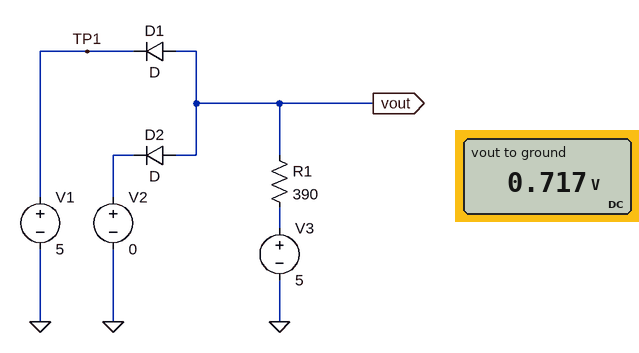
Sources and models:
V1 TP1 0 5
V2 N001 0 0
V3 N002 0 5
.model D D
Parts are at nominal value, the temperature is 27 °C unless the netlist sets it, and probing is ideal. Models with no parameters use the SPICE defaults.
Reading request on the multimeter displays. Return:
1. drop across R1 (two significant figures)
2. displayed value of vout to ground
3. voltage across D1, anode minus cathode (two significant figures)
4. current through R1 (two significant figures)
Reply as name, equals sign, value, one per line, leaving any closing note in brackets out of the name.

drop across R1 = 4.3 V
displayed value of vout to ground = 0.717 V
voltage across D1, anode minus cathode = -4.3 V
current through R1 = 11 mA
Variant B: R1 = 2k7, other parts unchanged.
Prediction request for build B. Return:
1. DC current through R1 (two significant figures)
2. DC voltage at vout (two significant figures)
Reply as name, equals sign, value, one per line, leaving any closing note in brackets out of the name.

DC current through R1 = 1.6 mA
DC voltage at vout = 670 mV
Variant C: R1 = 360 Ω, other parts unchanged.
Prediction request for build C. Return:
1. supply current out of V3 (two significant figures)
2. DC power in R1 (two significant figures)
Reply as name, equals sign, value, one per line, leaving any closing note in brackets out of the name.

supply current out of V3 = 12 mA
DC power in R1 = 51 mW
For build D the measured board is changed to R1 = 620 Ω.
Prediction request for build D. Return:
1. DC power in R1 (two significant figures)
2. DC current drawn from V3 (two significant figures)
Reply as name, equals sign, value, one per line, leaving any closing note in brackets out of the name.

DC power in R1 = 30 mW
DC current drawn from V3 = 6.9 mA
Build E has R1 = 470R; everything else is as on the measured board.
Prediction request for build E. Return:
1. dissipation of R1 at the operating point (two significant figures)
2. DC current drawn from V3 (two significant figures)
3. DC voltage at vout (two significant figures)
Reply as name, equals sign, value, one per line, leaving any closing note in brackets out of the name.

dissipation of R1 at the operating point = 39 mW
DC current drawn from V3 = 9.1 mA
DC voltage at vout = 710 mV
